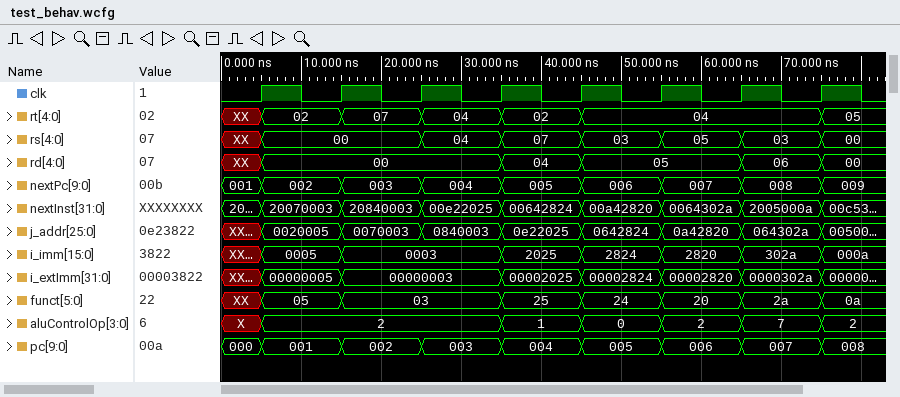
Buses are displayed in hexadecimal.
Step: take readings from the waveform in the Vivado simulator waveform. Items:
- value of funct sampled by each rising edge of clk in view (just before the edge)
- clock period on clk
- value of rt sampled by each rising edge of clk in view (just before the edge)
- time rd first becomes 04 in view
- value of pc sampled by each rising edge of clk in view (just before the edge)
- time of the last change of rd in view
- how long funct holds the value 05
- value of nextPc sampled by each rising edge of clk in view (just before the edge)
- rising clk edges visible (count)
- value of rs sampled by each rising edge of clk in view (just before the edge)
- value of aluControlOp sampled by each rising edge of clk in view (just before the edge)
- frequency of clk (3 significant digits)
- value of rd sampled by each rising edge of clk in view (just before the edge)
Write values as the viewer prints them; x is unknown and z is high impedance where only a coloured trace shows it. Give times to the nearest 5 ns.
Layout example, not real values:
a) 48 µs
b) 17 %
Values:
a) XX, 05, 03, 03, 25, 24, 20, 2a
b) 10 ns
c) XX, 02, 07, 04, 02, 04, 04, 04
d) 35 ns
e) 000, 001, 002, 003, 004, 005, 006, 007
f) 75 ns
g) 10 ns
h) 001, 002, 003, 004, 005, 006, 007, 008
i) 8
j) XX, 00, 00, 04, 07, 03, 05, 03
k) X, 2, 2, 2, 1, 0, 2, 7
l) 100 MHz
m) XX, 00, 00, 00, 04, 05, 05, 06
